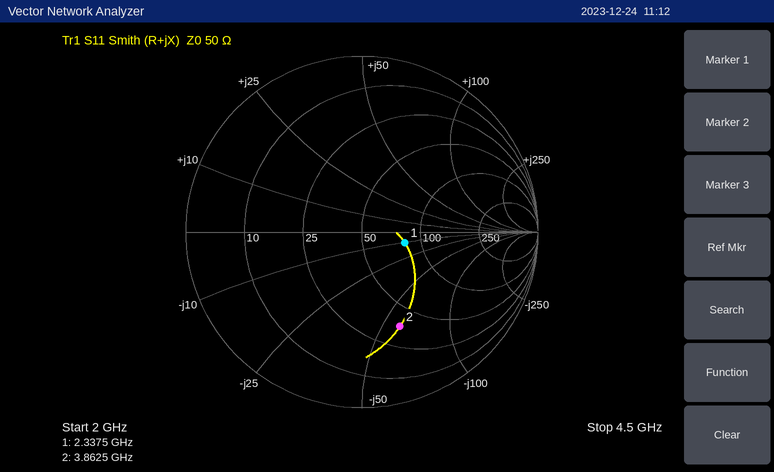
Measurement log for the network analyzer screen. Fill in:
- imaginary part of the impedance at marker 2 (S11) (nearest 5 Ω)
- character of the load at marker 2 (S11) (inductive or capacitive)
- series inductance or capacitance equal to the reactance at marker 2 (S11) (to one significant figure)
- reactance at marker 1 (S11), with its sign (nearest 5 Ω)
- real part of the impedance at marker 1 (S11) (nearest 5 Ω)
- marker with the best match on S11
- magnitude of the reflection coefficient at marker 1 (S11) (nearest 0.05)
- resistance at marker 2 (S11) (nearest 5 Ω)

-60 Ω
capacitive
700 fF
-10 Ω
80 Ω
marker 1
0.25
35 Ω
